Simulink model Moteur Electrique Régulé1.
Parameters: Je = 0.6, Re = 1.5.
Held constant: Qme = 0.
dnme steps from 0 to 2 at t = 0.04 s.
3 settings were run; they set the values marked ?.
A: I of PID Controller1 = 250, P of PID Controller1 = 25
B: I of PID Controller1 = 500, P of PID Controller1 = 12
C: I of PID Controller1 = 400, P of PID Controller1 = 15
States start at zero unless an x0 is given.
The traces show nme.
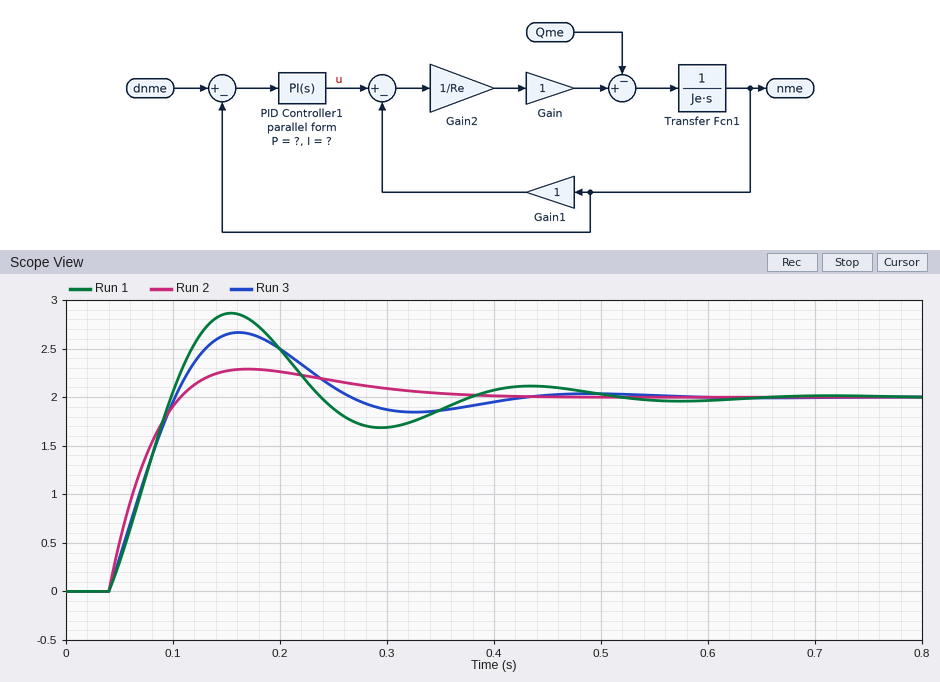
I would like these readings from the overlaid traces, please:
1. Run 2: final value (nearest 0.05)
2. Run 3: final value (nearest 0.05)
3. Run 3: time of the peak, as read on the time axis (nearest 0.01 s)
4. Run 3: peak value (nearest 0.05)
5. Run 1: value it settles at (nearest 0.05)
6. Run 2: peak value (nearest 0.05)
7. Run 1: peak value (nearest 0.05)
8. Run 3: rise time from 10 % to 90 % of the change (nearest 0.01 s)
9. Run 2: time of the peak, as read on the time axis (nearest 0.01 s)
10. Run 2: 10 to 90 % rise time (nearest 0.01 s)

2.00
2.00
0.16 s
2.65
2.00
2.30
2.85
0.05 s
0.17 s
0.05 s
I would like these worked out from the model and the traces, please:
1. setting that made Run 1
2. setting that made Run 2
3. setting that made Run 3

B
A
C
